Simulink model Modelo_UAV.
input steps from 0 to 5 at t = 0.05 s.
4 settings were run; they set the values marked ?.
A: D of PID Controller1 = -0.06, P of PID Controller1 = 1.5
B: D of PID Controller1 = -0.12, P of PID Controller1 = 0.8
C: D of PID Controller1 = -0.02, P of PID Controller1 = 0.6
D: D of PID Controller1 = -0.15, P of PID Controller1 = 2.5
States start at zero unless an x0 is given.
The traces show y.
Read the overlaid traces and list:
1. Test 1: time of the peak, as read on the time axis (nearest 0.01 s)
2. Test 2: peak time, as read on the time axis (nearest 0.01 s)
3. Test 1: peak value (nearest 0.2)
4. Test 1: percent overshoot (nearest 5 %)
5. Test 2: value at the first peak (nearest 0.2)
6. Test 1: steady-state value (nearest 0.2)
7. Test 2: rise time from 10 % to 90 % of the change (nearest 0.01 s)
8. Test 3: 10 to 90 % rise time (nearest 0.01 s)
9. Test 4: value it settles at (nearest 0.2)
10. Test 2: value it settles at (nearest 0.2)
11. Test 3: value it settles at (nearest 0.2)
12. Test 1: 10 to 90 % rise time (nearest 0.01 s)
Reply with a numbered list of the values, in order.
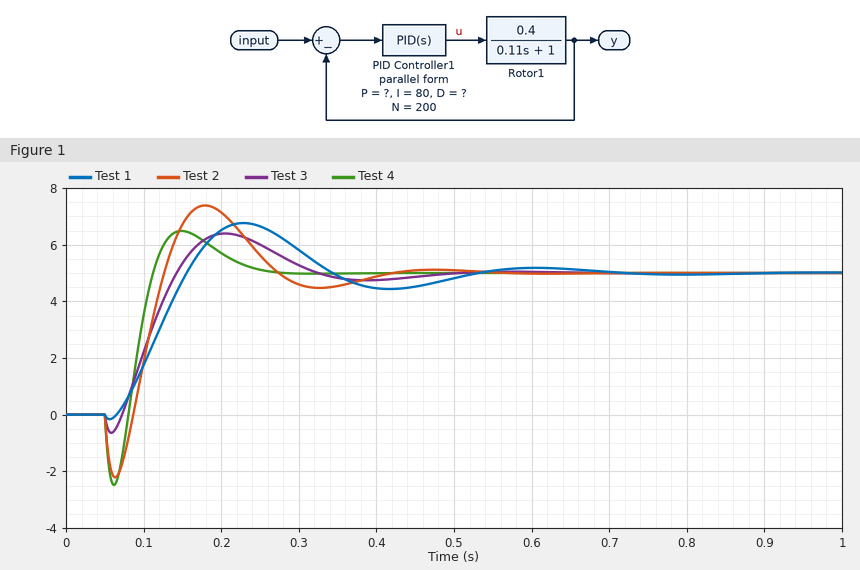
1. 0.23 s
2. 0.18 s
3. 6.8
4. 35 %
5. 7.4
6. 5.0
7. 0.03 s
8. 0.05 s
9. 5.0
10. 5.0
11. 5.0
12. 0.07 s
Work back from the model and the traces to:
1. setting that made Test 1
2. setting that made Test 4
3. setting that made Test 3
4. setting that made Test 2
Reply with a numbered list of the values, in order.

1. C
2. D
3. A
4. B
